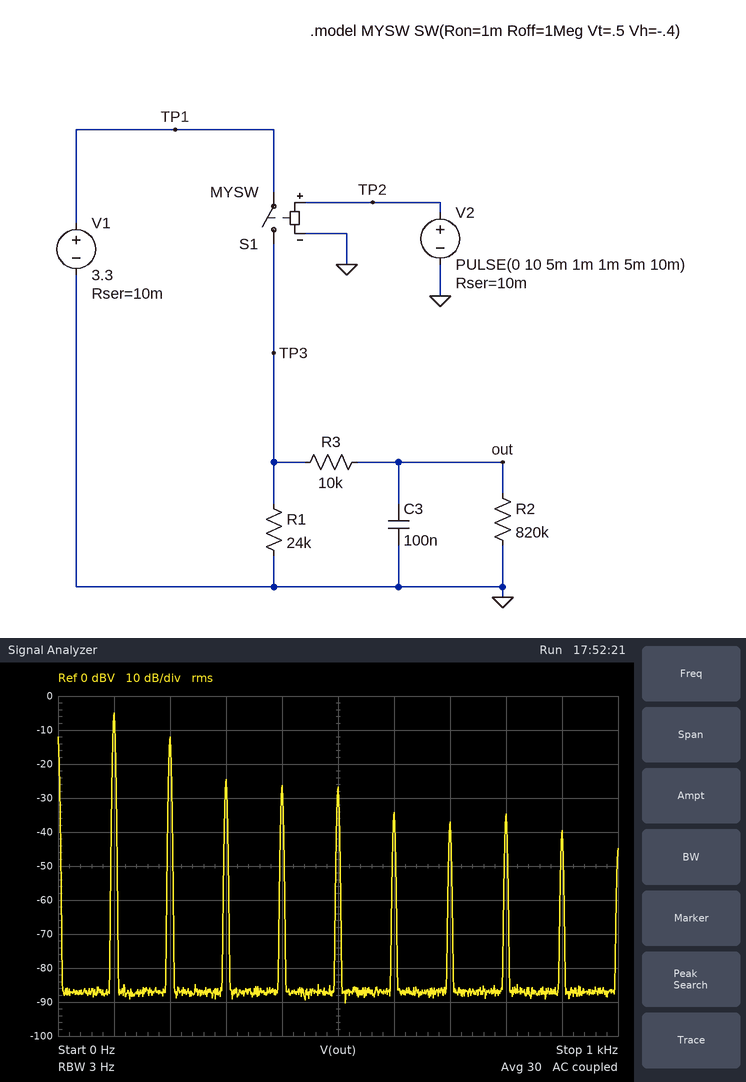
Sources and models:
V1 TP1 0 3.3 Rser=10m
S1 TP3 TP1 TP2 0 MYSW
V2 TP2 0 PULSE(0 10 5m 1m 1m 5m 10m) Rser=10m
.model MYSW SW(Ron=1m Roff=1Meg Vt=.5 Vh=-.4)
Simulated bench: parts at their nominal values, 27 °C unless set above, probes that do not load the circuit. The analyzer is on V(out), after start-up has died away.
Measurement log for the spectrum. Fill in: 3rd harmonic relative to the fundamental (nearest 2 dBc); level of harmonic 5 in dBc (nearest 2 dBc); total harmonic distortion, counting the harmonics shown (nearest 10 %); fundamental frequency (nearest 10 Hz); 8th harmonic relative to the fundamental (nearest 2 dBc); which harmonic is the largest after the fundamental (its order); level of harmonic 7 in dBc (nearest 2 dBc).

-20 dBc
-22 dBc
50 %
100 Hz
-30 dBc
2
-32 dBc
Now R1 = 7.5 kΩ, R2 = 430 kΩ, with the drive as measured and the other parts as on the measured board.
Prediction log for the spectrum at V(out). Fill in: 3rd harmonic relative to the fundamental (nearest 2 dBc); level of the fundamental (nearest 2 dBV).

-22 dBc
-2 dBV
